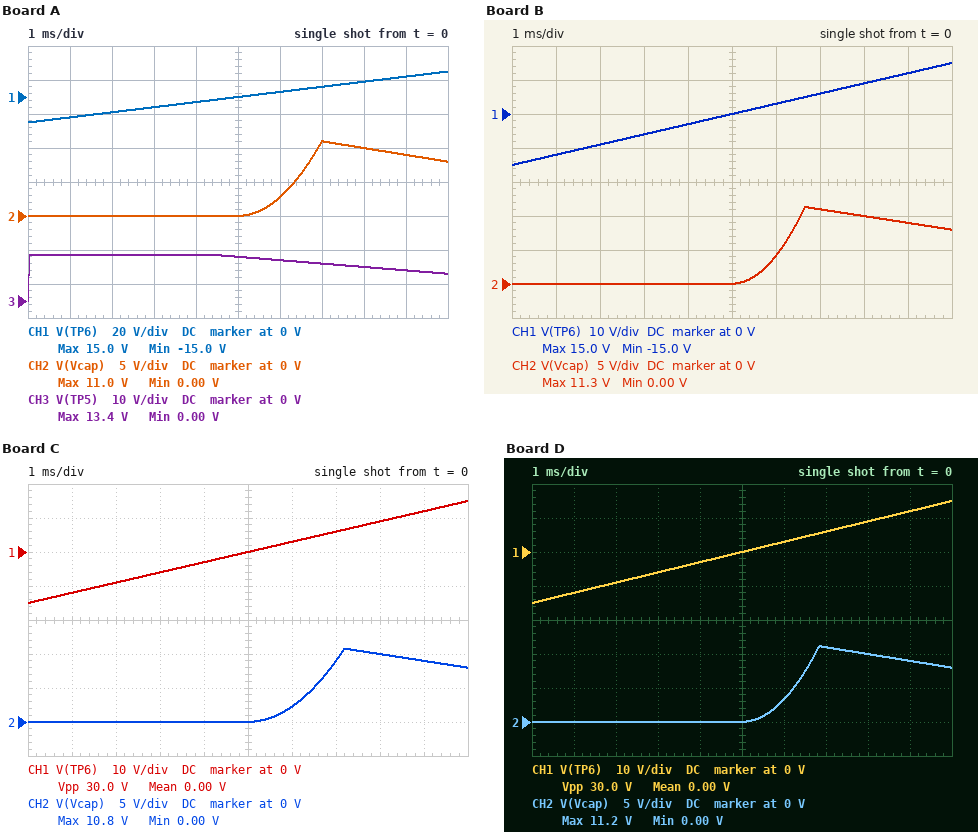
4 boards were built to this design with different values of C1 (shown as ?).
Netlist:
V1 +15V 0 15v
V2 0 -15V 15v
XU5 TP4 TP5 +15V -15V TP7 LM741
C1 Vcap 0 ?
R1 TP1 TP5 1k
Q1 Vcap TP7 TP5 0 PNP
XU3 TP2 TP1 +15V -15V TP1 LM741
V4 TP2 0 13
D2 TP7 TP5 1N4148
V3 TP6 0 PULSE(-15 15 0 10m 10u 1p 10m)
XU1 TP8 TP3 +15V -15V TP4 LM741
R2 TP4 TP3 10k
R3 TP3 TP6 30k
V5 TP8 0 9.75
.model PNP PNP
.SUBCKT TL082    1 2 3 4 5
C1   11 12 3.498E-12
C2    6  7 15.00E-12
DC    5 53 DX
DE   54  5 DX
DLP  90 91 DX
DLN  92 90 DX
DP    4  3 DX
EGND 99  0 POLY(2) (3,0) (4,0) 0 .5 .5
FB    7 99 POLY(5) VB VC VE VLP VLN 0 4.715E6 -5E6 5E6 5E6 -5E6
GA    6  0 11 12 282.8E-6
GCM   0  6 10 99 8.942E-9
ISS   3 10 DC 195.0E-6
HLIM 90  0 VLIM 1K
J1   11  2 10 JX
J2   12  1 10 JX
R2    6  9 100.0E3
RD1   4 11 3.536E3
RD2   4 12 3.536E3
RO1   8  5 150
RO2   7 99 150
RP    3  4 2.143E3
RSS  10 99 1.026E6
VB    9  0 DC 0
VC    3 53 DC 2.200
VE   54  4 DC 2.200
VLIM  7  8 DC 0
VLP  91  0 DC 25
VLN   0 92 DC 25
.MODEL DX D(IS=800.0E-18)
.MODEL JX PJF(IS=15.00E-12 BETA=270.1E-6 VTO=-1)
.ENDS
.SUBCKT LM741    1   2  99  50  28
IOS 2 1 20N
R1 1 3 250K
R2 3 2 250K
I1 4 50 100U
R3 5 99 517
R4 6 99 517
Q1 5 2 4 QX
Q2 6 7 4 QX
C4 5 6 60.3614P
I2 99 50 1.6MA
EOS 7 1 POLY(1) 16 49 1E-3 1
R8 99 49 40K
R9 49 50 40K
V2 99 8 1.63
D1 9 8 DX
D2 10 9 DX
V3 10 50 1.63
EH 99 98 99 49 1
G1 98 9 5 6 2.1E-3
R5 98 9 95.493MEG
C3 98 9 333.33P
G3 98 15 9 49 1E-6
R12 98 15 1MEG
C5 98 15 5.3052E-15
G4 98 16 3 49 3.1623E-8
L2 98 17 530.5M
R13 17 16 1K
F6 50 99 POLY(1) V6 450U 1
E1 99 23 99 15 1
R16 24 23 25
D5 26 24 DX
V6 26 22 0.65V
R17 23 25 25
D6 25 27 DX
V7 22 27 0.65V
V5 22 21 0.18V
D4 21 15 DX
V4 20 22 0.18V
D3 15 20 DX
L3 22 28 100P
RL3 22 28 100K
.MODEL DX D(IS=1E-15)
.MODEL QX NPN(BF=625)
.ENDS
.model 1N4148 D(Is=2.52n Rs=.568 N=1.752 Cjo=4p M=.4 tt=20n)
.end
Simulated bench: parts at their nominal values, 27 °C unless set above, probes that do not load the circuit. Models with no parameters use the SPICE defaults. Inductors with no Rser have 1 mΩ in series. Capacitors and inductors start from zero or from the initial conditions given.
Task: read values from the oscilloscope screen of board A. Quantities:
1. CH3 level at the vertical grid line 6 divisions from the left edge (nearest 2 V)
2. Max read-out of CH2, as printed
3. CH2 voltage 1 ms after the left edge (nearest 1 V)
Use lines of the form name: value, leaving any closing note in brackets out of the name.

CH3 level at the vertical grid line 6 divisions from the left edge: 12 V
Max read-out of CH2, as printed: 11.0 V
CH2 voltage 1 ms after the left edge: 0 V
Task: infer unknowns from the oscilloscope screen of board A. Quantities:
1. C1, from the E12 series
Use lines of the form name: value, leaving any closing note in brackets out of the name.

C1, from the E12 series: 180 nF
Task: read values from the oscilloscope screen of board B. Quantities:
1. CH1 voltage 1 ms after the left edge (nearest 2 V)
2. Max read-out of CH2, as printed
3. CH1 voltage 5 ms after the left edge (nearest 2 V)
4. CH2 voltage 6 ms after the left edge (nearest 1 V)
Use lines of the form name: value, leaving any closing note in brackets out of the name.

CH1 voltage 1 ms after the left edge: -12 V
Max read-out of CH2, as printed: 11.3 V
CH1 voltage 5 ms after the left edge: 0 V
CH2 voltage 6 ms after the left edge: 4 V
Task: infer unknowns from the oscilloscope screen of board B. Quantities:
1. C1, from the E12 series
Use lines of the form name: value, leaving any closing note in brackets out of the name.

C1, from the E12 series: 120 nF
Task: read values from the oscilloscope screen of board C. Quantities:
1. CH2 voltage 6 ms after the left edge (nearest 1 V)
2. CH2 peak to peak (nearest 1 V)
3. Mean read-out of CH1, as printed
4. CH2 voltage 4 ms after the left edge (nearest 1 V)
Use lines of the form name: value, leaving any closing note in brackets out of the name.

CH2 voltage 6 ms after the left edge: 2 V
CH2 peak to peak: 11 V
Mean read-out of CH1, as printed: 0.00 V
CH2 voltage 4 ms after the left edge: 0 V
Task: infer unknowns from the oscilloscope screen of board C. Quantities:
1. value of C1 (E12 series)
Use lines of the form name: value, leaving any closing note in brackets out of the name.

value of C1: 220 nF
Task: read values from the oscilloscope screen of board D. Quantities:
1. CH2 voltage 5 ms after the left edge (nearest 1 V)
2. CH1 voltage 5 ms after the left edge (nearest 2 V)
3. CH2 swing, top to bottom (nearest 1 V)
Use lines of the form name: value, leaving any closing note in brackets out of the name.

CH2 voltage 5 ms after the left edge: 0 V
CH1 voltage 5 ms after the left edge: 0 V
CH2 swing, top to bottom: 11 V
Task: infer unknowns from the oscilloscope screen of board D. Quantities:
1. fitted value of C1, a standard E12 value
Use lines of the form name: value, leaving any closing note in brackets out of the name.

fitted value of C1, a standard E12 value: 150 nF
